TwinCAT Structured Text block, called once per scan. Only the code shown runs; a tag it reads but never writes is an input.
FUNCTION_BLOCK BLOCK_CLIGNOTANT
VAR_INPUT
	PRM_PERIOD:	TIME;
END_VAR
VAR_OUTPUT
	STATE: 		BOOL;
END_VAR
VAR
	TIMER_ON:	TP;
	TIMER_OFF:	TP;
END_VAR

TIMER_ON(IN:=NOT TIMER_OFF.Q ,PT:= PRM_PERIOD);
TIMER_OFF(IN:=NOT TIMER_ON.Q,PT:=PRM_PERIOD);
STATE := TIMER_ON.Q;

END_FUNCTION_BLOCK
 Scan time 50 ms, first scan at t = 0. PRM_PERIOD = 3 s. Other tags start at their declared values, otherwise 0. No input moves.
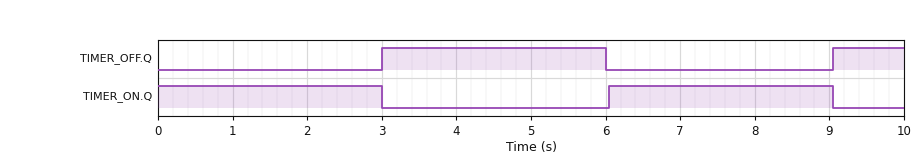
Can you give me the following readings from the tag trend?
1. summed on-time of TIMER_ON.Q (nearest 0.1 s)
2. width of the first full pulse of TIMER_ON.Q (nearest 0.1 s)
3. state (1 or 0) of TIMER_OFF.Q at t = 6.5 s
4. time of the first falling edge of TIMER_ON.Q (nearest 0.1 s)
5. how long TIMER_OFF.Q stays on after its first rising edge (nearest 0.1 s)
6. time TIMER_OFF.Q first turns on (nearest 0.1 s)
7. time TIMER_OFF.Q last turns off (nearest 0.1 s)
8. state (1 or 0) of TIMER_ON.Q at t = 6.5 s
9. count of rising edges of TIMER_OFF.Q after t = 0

6.0 s
3.0 s
0
3.0 s
3.0 s
3.0 s
6.0 s
1
2
